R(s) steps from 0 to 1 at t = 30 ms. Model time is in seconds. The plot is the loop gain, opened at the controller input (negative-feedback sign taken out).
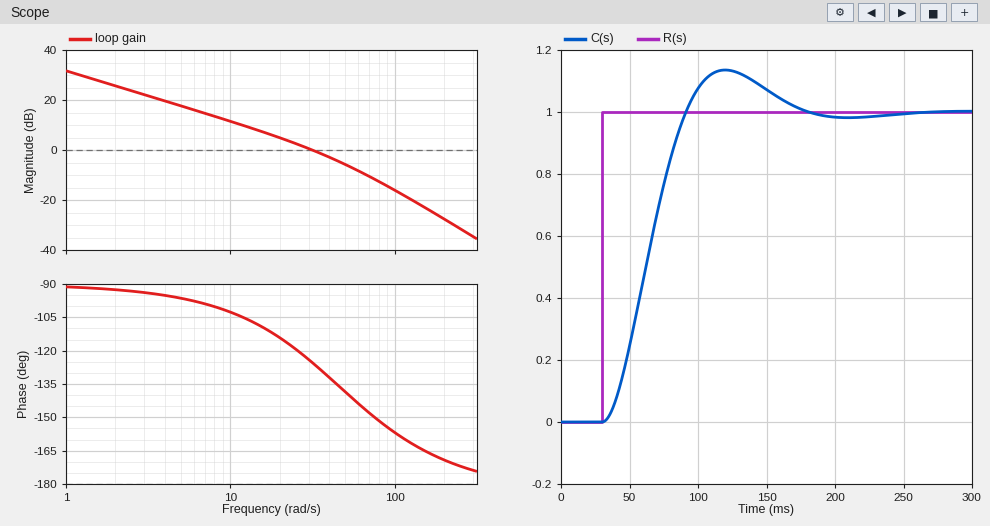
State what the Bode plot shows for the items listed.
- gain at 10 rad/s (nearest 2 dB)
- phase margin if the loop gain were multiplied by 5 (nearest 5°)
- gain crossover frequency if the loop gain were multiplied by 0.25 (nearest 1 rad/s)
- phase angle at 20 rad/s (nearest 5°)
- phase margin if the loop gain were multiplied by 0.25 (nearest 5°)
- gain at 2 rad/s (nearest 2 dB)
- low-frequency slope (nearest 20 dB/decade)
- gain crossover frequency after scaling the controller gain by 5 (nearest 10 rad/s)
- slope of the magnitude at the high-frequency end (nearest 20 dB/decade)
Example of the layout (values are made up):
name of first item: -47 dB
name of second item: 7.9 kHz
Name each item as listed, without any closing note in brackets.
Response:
gain at 10 rad/s: 12 dB
phase margin if the loop gain were multiplied by 5: 25°
gain crossover frequency if the loop gain were multiplied by 0.25: 9 rad/s
phase angle at 20 rad/s: -115°
phase margin if the loop gain were multiplied by 0.25: 80°
gain at 2 rad/s: 26 dB
low-frequency slope: -20 dB/decade
gain crossover frequency after scaling the controller gain by 5: 90 rad/s
slope of the magnitude at the high-frequency end: -40 dB/decade
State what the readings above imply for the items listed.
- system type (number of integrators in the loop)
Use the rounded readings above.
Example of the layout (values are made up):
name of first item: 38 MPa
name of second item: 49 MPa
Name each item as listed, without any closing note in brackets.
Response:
system type: 1
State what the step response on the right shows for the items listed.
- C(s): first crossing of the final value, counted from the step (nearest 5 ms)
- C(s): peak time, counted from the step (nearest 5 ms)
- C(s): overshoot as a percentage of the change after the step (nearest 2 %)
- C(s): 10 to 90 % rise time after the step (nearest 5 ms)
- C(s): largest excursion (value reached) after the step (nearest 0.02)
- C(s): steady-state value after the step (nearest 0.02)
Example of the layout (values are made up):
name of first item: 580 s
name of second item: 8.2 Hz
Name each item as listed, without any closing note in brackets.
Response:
C(s): first crossing of the final value, counted from the step: 60 ms
C(s): peak time, counted from the step: 90 ms
C(s): overshoot as a percentage of the change after the step: 14 %
C(s): 10 to 90 % rise time after the step: 40 ms
C(s): largest excursion (value reached) after the step: 1.14
C(s): steady-state value after the step: 1.00
